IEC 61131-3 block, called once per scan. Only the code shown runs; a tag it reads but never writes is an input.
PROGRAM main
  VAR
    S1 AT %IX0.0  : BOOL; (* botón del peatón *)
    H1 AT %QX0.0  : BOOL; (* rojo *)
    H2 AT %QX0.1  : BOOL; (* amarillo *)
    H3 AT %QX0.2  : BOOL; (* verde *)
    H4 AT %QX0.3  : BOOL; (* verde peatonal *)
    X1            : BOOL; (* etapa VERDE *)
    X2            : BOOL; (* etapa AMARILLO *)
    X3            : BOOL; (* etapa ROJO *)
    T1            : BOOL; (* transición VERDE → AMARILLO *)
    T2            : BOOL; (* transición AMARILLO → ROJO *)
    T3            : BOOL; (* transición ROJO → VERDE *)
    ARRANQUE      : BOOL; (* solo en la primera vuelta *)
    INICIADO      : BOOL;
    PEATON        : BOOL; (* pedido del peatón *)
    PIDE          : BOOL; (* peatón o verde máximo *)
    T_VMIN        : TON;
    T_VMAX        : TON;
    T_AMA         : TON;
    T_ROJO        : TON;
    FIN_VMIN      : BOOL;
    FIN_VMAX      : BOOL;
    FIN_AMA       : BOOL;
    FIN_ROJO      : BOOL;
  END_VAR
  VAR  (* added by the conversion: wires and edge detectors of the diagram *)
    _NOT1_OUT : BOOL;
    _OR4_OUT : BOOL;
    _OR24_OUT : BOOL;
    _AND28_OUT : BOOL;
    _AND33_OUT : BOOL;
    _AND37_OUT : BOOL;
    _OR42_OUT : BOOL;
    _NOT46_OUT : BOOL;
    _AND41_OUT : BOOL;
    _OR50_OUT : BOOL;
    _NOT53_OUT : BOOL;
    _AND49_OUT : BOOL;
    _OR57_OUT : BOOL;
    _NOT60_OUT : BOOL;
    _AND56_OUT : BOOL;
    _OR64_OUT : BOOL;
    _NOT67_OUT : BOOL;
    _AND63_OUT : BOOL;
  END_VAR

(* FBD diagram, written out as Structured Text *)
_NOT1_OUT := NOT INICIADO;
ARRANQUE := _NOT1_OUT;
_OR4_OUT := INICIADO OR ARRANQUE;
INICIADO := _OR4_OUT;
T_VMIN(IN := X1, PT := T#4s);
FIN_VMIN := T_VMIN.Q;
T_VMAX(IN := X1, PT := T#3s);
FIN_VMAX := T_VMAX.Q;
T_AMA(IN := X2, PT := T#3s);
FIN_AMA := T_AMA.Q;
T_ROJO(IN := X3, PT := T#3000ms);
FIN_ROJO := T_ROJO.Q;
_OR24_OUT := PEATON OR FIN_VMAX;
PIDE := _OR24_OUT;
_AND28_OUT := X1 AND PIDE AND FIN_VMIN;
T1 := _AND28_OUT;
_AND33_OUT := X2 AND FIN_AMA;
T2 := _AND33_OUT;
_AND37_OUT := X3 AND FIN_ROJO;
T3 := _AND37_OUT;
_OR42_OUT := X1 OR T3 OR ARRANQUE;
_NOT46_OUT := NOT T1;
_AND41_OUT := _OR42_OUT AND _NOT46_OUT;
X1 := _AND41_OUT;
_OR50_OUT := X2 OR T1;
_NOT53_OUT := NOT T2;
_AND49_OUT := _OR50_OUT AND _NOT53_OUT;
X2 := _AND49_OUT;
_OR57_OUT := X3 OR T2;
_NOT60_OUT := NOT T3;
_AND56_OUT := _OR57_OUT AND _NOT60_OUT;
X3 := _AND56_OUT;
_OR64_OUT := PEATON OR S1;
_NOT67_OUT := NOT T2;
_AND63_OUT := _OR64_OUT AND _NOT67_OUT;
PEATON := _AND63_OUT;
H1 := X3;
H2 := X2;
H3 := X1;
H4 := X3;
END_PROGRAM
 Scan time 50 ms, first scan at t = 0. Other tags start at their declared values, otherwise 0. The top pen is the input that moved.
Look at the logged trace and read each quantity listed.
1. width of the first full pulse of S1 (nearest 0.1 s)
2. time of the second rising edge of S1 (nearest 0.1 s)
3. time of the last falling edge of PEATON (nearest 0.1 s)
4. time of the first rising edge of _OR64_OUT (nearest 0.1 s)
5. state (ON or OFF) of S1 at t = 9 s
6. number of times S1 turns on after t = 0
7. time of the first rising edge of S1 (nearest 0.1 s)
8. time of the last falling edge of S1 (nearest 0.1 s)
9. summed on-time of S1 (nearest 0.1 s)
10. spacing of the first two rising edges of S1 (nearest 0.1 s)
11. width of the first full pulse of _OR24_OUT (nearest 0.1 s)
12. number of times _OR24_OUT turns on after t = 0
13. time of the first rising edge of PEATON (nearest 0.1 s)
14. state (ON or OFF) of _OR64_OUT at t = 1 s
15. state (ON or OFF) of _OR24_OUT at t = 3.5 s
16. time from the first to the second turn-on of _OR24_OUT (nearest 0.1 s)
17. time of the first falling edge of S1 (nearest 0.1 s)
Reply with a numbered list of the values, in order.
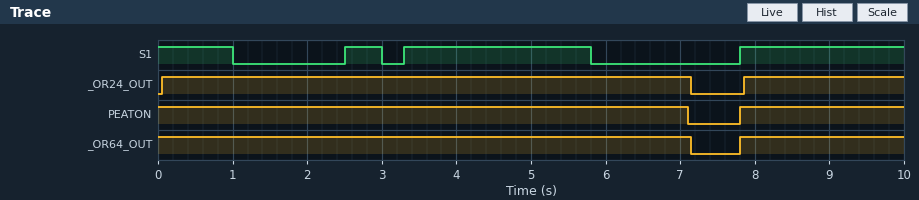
1. 0.5 s
2. 3.3 s
3. 7.1 s
4. 7.8 s
5. ON
6. 3
7. 2.5 s
8. 5.8 s
9. 6.2 s
10. 0.8 s
11. 7.1 s
12. 2
13. 7.8 s
14. ON
15. ON
16. 7.8 s
17. 1.0 s
